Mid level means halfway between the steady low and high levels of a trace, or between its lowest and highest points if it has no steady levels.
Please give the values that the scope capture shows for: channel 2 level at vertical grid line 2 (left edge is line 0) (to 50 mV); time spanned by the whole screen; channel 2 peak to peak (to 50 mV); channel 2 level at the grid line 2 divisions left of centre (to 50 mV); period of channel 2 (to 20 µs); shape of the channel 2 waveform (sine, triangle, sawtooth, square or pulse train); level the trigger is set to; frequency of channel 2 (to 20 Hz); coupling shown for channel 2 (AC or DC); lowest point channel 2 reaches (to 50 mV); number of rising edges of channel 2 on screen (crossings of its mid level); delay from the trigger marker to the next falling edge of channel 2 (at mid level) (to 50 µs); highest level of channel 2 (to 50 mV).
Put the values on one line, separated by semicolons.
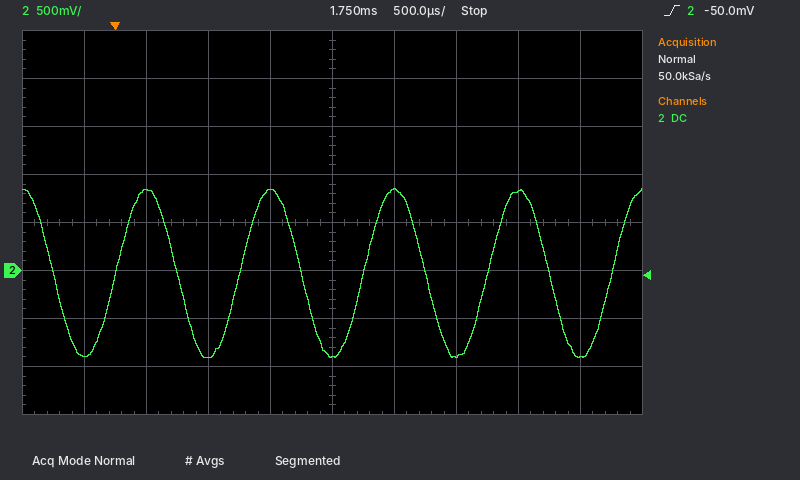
850 mV; 5 ms; 1.75 V; -900 mV; 1.00 ms; sine; -50.0 mV; 1.00 kHz; DC; -900 mV; 5; 500 µs; 850 mV
